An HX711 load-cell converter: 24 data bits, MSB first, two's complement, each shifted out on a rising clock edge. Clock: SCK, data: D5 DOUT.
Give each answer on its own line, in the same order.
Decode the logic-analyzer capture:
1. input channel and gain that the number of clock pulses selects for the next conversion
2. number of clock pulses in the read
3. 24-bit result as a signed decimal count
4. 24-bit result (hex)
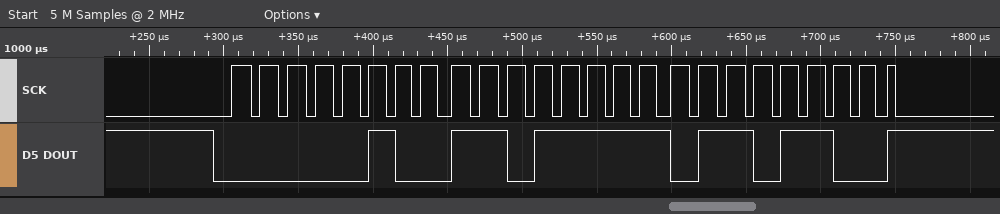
channel A, gain 128
25
319340
0x04DF6C
